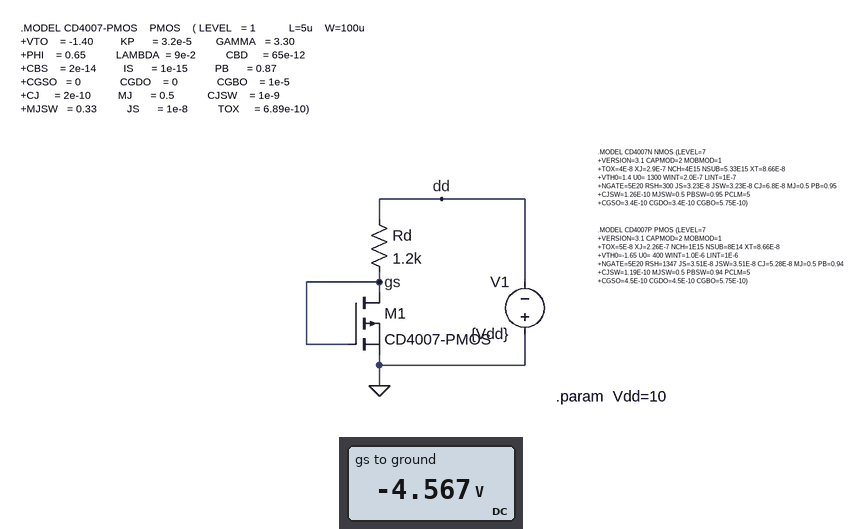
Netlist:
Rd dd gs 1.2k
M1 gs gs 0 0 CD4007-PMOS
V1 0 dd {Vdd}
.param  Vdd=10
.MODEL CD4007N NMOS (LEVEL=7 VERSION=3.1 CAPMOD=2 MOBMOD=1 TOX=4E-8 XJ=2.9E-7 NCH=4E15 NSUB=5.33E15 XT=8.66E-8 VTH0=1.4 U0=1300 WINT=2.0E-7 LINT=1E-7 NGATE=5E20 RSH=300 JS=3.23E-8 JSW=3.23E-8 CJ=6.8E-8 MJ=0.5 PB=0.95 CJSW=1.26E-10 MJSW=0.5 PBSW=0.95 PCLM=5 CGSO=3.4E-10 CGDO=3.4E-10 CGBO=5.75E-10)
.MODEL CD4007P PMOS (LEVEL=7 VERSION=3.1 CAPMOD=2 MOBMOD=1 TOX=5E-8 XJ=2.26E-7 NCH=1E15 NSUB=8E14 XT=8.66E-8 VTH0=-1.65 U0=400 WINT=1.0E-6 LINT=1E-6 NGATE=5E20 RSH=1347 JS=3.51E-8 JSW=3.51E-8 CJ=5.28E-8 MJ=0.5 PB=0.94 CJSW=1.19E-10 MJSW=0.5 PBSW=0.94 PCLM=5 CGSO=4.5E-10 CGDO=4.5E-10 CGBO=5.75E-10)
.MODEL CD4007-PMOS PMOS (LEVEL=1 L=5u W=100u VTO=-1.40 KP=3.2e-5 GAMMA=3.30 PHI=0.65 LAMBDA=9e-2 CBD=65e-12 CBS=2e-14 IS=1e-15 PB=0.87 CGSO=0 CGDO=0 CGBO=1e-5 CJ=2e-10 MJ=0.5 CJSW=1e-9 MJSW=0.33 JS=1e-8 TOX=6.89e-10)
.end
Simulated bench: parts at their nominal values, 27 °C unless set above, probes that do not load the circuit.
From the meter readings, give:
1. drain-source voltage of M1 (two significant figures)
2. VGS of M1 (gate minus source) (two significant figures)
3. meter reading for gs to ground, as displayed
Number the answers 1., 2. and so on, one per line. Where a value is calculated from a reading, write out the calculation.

1. -4.567 V = -4.6 V
2. -4.567 V = -4.6 V
3. -4.567 V
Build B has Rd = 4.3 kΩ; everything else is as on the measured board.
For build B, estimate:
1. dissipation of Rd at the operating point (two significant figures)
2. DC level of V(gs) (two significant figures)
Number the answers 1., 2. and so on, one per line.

1. 10 mW
2. -3.3 V
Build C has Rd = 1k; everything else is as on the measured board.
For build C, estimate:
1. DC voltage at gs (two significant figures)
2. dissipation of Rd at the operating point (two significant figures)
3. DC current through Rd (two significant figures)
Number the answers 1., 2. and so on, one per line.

1. -4.8 V
2. 27 mW
3. 5.2 mA
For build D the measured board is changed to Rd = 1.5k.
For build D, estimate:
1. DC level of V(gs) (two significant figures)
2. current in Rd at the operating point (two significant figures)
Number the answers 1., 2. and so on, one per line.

1. -4.3 V
2. 3.8 mA
